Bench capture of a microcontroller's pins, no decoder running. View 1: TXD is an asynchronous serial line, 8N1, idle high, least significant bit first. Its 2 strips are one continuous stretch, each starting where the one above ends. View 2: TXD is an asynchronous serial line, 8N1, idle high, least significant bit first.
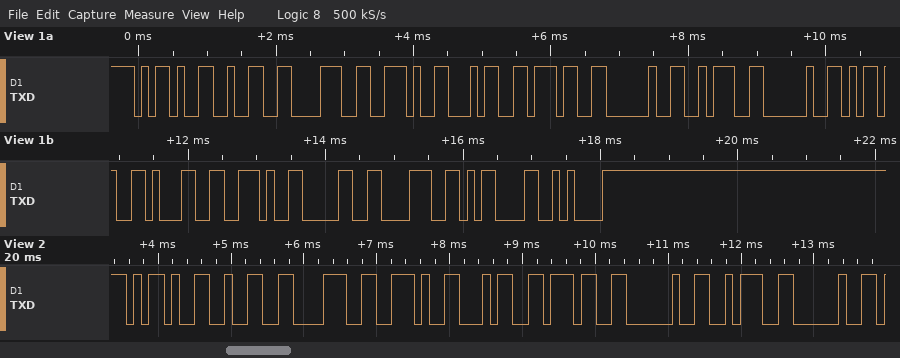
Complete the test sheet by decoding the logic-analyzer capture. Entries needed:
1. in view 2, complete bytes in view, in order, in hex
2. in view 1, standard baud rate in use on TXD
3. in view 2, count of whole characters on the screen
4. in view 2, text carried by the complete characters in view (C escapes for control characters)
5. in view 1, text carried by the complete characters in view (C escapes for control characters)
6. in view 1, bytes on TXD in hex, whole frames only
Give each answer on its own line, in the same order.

2D 32 38 2E 34 37 20 3A 20
9600 baud
9
"-28.47 : "
"-28.47 : -1.08\r\n"
2D 32 38 2E 34 37 20 3A 20 2D 31 2E 30 38 0D 0A
